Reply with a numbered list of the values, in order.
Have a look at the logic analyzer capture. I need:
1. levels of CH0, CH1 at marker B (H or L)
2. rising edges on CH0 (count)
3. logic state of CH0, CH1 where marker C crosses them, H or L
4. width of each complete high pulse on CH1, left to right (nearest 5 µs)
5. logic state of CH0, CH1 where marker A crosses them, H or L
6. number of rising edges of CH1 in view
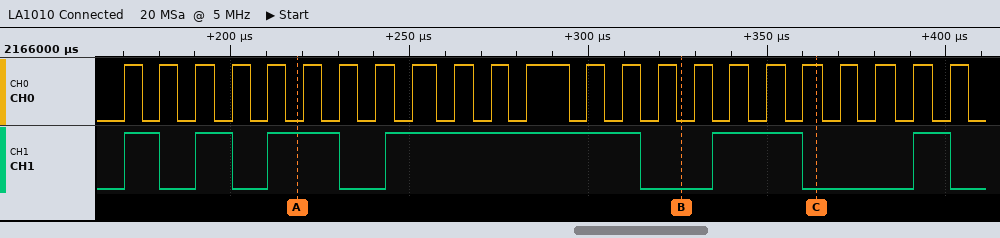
1. CH0=L, CH1=L
2. 23
3. CH0=H, CH1=L
4. 10 µs, 10 µs, 20 µs, 70 µs, 25 µs, 10 µs
5. CH0=L, CH1=H
6. 6
